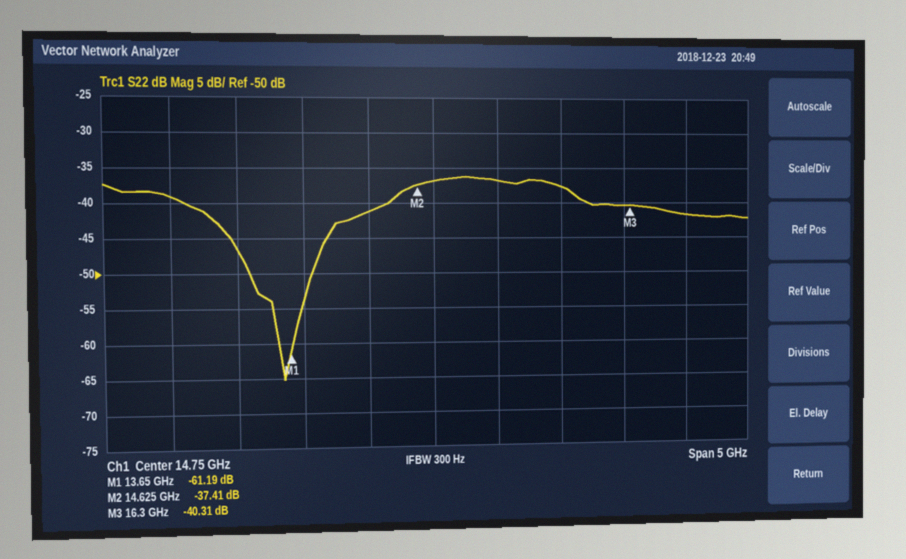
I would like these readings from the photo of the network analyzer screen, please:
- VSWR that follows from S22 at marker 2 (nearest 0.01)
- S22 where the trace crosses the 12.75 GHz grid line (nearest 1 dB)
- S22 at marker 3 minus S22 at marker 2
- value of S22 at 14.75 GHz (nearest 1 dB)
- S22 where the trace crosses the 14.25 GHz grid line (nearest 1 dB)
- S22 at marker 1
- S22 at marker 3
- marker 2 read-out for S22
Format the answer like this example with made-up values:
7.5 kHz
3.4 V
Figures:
1.03
-39 dB
-2.90 dB
-37 dB
-41 dB
-61.19 dB
-40.31 dB
-37.41 dB
